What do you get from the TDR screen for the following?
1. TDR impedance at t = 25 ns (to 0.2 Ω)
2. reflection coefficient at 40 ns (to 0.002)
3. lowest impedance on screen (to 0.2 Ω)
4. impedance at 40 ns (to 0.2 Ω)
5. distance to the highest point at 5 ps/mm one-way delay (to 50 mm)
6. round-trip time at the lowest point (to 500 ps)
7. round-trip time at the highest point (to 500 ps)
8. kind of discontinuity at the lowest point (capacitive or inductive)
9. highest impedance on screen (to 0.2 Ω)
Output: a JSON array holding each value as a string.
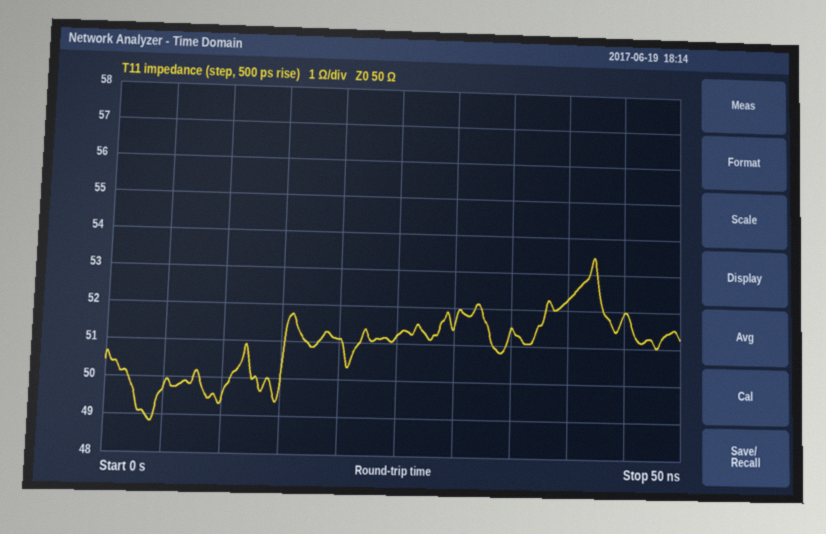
["51.2 Ω", "+0.022", "48.8 Ω", "52.2 Ω", "4.25 m", "4.0 ns", "42.5 ns", "capacitive", "53.4 Ω"]
